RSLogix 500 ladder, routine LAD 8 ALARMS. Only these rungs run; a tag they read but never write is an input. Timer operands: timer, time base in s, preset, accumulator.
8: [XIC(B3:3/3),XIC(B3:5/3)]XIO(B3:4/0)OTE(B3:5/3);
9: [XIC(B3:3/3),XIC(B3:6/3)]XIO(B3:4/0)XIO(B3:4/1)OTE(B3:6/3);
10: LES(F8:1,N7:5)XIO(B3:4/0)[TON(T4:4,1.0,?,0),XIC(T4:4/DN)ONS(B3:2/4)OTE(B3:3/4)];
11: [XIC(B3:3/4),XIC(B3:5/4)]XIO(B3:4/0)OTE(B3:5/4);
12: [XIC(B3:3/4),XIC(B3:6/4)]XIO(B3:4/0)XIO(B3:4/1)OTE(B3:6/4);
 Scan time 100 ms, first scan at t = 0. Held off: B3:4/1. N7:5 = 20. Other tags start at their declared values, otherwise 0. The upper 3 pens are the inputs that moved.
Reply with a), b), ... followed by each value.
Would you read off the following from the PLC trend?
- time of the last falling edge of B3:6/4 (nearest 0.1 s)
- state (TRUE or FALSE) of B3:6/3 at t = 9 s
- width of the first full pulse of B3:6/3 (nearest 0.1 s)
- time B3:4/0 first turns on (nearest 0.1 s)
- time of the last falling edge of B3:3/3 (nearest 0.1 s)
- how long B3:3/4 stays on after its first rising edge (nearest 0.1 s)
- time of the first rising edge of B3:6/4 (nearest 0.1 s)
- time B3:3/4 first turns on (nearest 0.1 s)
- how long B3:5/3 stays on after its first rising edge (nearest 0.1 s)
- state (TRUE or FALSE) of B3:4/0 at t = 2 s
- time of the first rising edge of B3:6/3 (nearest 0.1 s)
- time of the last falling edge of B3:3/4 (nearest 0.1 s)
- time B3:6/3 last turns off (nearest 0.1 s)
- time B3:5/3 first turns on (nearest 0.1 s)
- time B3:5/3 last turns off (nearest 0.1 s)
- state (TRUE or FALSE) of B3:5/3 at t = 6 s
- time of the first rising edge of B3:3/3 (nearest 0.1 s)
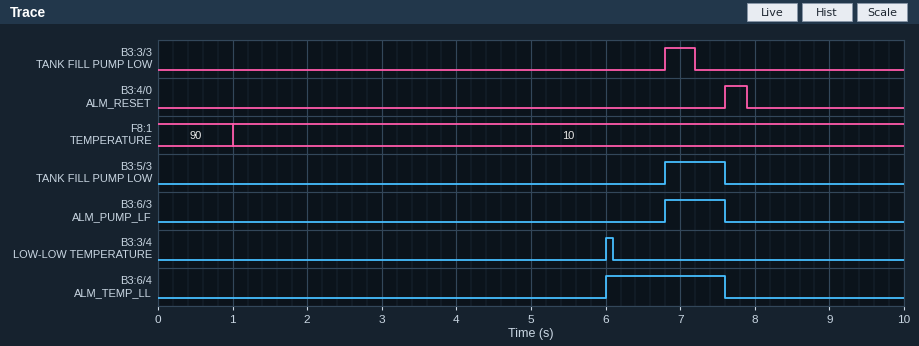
a) 7.6 s
b) FALSE
c) 0.8 s
d) 7.6 s
e) 7.2 s
f) 0.1 s
g) 6.0 s
h) 6.0 s
i) 0.8 s
j) FALSE
k) 6.8 s
l) 6.1 s
m) 7.6 s
n) 6.8 s
o) 7.6 s
p) FALSE
q) 6.8 s
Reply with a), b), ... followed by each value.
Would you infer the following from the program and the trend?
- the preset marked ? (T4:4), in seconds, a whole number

a) 5 s
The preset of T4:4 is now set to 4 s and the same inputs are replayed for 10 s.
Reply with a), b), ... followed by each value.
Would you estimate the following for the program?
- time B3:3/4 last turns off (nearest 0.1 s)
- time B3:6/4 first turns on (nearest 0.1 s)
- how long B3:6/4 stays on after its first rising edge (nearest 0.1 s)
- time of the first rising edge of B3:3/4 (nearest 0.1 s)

a) 5.1 s
b) 5.0 s
c) 2.6 s
d) 5.0 s
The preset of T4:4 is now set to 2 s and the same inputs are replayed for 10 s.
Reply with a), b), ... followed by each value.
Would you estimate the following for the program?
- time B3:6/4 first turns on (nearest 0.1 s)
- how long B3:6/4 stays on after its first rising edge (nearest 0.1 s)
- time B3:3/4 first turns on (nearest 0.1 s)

a) 3.0 s
b) 4.6 s
c) 3.0 s
